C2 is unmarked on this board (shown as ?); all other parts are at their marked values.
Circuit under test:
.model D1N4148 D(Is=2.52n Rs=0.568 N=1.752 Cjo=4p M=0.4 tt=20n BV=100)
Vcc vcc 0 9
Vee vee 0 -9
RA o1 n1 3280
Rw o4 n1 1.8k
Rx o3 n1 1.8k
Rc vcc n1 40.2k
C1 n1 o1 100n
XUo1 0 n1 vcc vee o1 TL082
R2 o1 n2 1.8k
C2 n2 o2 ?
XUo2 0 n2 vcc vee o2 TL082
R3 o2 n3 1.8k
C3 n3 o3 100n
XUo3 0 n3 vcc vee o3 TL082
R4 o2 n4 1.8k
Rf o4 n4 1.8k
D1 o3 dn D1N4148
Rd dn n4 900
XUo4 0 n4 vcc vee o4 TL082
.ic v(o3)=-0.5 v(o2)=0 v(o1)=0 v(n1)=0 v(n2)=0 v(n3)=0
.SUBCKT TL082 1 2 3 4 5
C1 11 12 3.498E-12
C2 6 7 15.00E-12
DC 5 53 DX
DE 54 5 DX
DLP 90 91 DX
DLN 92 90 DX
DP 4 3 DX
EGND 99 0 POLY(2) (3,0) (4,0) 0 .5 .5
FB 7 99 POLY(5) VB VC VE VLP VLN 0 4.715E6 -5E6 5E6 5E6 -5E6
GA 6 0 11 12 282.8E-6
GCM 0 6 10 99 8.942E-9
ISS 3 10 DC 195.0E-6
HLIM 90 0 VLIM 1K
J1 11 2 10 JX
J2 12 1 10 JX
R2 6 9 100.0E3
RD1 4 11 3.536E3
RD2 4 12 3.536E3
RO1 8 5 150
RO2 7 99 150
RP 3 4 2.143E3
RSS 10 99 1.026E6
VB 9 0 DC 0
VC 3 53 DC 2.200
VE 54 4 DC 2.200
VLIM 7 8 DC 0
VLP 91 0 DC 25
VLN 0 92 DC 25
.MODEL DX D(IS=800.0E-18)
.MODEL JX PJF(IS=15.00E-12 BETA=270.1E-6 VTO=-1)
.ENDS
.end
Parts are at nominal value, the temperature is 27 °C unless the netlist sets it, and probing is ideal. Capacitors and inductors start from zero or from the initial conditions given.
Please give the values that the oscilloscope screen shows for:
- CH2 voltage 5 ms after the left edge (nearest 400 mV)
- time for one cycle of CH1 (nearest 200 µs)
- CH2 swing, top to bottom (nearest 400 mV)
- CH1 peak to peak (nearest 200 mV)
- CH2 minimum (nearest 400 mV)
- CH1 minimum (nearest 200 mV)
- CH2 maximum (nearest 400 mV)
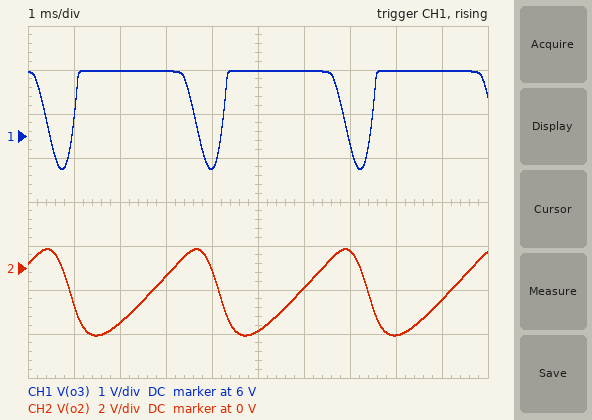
-2.8 V
3.2 ms
4.0 V
2.2 V
-3.2 V
5.2 V
800 mV
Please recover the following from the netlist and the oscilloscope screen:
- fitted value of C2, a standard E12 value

180 nF
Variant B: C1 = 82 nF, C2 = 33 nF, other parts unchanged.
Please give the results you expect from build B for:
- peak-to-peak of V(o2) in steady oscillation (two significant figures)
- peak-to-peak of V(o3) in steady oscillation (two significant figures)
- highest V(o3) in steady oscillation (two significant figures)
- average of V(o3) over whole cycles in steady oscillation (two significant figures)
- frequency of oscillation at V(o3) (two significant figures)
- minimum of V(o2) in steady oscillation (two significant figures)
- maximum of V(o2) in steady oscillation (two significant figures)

4.9 V
2.6 V
1.1 V
-160 mV
1.7 kHz
-2.6 V
2.4 V
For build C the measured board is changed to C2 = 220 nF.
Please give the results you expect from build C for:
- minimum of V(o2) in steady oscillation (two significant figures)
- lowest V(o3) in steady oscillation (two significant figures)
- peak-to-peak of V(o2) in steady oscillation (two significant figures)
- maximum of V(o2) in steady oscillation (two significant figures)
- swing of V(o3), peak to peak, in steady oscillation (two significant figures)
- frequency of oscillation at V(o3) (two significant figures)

-2.5 V
5.4 V
3.2 V
730 mV
2.1 V
300 Hz
